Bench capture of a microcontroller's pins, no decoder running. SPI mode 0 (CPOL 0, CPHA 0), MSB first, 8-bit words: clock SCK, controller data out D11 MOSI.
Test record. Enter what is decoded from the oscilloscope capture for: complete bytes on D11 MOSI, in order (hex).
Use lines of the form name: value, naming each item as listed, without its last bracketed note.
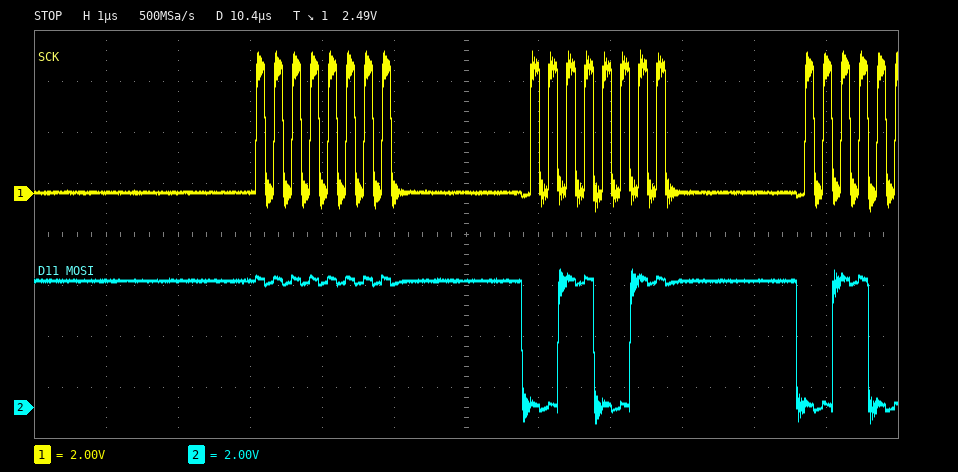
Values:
complete bytes on D11 MOSI, in order: 0xFF 0x33
